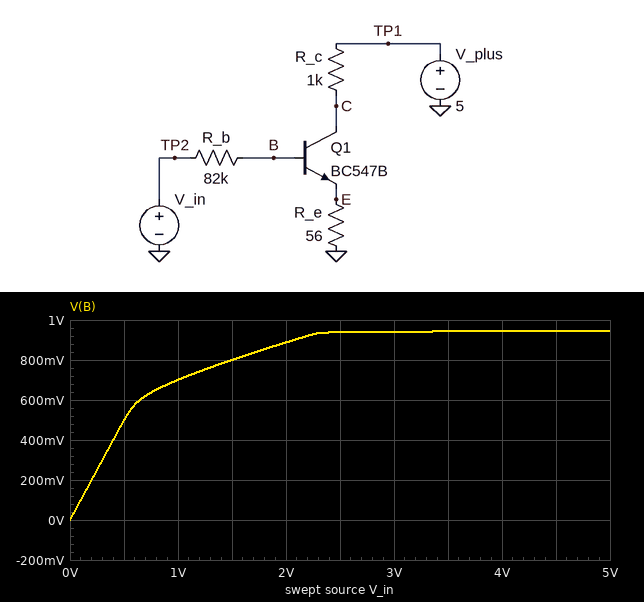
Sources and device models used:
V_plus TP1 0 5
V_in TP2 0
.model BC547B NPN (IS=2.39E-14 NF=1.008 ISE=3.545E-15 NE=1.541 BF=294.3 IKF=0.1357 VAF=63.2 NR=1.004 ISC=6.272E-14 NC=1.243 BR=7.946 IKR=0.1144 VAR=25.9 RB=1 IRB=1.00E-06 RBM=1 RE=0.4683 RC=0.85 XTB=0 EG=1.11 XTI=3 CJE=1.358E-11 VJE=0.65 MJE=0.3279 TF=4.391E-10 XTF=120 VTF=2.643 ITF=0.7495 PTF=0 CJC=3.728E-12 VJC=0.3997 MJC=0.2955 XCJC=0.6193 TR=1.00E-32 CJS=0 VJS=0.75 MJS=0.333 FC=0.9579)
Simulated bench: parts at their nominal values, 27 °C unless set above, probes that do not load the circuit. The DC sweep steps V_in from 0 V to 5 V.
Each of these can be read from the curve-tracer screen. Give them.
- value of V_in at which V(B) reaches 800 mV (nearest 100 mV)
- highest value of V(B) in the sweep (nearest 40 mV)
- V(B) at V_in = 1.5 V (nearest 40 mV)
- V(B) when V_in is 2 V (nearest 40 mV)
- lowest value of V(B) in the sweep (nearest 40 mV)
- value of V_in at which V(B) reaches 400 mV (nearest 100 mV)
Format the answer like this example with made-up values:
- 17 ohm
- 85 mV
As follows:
- 1.5 V
- 960 mV
- 800 mV
- 880 mV
- 0 V
- 400 mV
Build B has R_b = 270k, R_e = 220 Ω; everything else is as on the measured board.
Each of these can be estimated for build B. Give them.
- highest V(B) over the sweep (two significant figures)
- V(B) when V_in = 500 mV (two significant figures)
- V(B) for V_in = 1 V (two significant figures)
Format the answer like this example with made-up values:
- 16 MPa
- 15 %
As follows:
- 1.5 V
- 500 mV
- 690 mV
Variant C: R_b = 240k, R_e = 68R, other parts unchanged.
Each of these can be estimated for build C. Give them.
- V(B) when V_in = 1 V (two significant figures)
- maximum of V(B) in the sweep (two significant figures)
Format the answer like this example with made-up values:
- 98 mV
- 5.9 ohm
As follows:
- 650 mV
- 990 mV
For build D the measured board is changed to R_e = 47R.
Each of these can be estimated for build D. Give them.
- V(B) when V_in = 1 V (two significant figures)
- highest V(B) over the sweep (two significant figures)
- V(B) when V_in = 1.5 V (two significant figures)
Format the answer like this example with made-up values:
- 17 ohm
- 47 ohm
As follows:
- 690 mV
- 910 mV
- 780 mV
